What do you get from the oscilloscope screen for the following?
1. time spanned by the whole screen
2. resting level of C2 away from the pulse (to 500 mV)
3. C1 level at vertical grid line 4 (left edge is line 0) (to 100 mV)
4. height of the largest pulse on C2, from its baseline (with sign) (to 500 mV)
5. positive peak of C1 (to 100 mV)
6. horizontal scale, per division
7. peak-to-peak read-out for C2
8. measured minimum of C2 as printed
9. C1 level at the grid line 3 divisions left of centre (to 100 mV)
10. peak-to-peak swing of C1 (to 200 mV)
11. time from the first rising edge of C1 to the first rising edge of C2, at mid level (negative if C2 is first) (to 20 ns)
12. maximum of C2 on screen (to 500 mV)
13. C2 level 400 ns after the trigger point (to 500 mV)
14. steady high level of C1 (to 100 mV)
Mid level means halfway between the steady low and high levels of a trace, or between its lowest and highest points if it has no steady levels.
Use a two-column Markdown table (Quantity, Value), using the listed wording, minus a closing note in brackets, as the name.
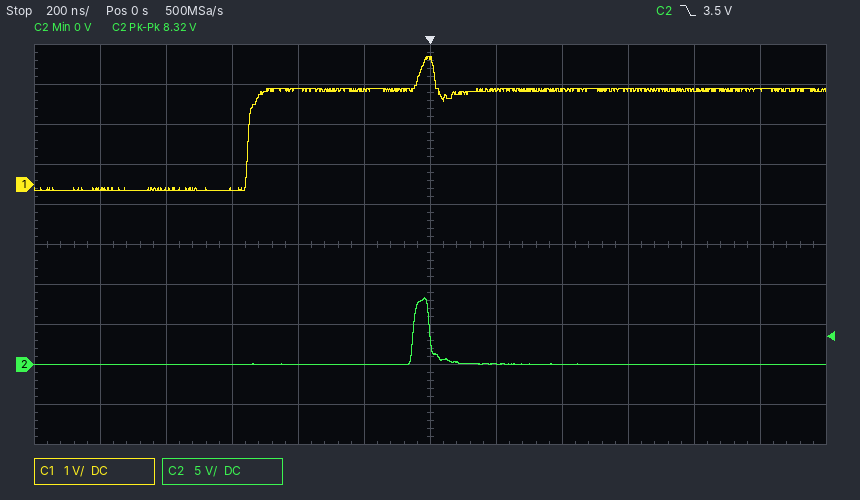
| Quantity | Value |
|---|---|
| time spanned by the whole screen | 2.4 µs |
| resting level of C2 away from the pulse | 0.0 V |
| C1 level at vertical grid line 4 (left edge is line 0) | 2.4 V |
| height of the largest pulse on C2, from its baseline (with sign) | +8.5 V |
| positive peak of C1 | 3.2 V |
| horizontal scale, per division | 200 ns |
| peak-to-peak read-out for C2 | 8.32 V |
| measured minimum of C2 as printed | 0 V |
| C1 level at the grid line 3 divisions left of centre | -100 mV |
| peak-to-peak swing of C1 | 3.4 V |
| time from the first rising edge of C1 to the first rising edge of C2, at mid level (negative if C2 is first) | +500 ns |
| maximum of C2 on screen | 8.5 V |
| C2 level 400 ns after the trigger point | 0.0 V |
| steady high level of C1 | 2.4 V |
